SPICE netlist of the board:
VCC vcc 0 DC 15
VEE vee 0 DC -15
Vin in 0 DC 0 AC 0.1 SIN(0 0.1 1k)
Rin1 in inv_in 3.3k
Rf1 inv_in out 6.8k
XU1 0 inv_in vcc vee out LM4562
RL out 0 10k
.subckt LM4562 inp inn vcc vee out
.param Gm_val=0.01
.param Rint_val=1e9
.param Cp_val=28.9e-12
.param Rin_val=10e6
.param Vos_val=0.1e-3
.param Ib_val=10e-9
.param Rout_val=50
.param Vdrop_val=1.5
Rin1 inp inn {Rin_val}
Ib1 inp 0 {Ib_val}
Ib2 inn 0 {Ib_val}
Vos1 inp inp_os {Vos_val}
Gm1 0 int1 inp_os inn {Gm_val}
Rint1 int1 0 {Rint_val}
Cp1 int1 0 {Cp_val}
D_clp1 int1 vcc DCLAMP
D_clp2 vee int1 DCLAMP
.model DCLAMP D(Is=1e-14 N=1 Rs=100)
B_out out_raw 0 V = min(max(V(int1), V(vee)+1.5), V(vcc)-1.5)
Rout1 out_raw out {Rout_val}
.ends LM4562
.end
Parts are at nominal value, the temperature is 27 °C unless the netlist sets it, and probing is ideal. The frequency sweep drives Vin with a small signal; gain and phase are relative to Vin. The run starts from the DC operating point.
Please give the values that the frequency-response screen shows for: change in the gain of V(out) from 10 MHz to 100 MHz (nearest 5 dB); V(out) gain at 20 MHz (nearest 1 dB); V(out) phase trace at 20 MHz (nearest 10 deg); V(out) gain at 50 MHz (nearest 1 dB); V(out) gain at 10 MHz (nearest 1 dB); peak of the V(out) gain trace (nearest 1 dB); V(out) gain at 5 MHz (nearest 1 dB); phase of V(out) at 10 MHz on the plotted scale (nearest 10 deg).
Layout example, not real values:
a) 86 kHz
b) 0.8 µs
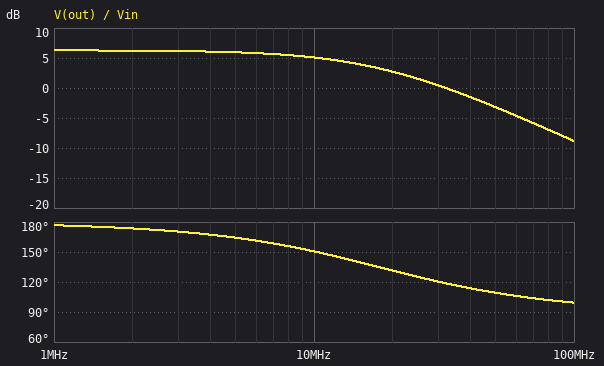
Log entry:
a) -15 dB
b) 3 dB
c) 130 deg
d) -3 dB
e) 5 dB
f) 6 dB
g) 6 dB
h) 150 deg
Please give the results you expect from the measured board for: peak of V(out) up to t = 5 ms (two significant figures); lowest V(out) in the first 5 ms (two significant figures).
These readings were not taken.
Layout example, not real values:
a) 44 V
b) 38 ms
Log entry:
a) 210 mV
b) -210 mV
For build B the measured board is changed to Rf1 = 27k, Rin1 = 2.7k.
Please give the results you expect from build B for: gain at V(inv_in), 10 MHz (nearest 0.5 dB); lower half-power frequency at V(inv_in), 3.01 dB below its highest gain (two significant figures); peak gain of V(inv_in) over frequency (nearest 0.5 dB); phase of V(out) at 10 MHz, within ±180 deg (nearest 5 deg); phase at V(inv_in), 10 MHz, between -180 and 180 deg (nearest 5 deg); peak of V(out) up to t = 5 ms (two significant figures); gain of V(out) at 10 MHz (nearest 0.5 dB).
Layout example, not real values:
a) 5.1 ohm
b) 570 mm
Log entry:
a) -2.0 dB
b) 5.0 MHz
c) -1.0 dB
d) 115 deg
e) 25 deg
f) 1.0 V
g) 13.0 dB
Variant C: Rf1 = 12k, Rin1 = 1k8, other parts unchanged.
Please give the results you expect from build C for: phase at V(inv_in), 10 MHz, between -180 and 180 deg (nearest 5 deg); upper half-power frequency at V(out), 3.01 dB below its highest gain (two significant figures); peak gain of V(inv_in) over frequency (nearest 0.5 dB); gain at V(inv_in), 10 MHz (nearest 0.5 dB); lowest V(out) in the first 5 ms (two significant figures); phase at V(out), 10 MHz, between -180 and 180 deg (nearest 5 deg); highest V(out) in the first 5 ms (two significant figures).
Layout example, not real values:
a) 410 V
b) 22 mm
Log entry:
a) 35 deg
b) 7.1 MHz
c) -1.0 dB
d) -3.0 dB
e) -670 mV
f) 125 deg
g) 670 mV
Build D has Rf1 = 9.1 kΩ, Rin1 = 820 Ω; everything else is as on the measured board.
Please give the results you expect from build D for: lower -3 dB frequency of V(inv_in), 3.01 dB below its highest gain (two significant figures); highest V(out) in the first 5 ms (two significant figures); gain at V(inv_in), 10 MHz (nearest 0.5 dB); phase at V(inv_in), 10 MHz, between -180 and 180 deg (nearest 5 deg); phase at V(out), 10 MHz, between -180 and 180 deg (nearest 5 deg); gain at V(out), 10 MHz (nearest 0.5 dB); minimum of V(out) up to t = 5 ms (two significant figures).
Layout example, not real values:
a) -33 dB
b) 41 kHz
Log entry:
a) 4.5 MHz
b) 1.1 V
c) -1.5 dB
d) 25 deg
e) 115 deg
f) 13.0 dB
g) -1.1 V
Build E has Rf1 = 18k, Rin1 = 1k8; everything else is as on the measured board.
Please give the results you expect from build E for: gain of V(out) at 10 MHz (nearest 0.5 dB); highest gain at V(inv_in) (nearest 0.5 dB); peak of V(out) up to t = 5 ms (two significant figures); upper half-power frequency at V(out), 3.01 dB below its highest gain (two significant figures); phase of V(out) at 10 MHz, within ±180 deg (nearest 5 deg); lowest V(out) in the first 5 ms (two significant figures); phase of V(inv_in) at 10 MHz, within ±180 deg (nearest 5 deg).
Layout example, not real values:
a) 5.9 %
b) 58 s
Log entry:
a) 13.0 dB
b) -1.0 dB
c) 1.0 V
d) 5.0 MHz
e) 115 deg
f) -1.0 V
g) 25 deg
